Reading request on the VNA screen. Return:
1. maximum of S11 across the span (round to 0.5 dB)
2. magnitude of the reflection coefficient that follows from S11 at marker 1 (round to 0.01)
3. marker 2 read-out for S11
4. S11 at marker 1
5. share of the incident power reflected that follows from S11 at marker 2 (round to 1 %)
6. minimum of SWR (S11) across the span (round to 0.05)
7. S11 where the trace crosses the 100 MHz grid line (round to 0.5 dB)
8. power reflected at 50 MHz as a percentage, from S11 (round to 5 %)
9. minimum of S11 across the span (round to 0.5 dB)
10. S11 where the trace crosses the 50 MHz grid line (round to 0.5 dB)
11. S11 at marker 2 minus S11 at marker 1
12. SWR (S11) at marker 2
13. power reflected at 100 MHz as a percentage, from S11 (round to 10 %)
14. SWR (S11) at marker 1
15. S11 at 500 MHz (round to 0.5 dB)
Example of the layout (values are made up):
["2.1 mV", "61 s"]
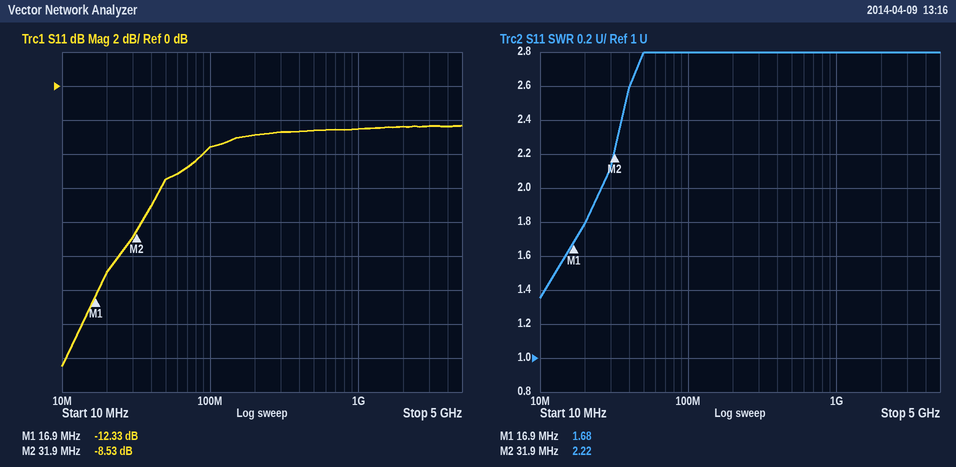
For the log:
["-2.5 dB", "0.24", "-8.53 dB", "-12.33 dB", "14 %", "1.35", "-3.5 dB", "30 %", "-16.5 dB", "-5.5 dB", "3.80 dB", "2.22", "40 %", "1.68", "-2.5 dB"]
